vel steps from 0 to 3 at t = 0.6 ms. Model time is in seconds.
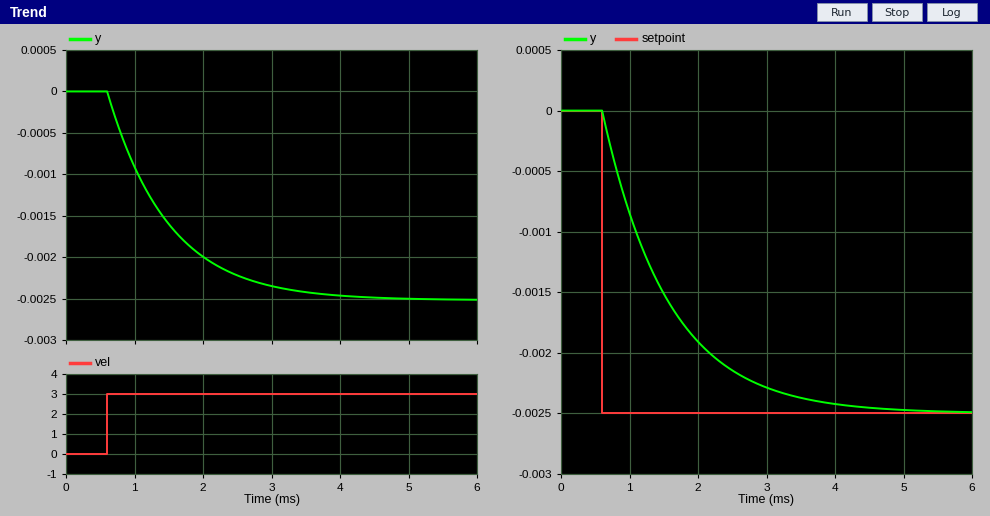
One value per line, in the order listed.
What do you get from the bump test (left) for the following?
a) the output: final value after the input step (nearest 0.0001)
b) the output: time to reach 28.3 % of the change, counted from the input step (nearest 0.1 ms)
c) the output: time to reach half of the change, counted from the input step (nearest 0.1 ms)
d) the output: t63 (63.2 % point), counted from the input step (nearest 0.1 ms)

-0.0025
0.3 ms
0.6 ms
0.9 ms
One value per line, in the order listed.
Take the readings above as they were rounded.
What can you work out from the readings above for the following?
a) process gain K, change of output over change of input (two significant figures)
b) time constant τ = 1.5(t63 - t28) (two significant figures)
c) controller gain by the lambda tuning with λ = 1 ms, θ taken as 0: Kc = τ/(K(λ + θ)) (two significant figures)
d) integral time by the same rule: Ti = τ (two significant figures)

-0.00083
0.90 ms
-1100
0.90 ms
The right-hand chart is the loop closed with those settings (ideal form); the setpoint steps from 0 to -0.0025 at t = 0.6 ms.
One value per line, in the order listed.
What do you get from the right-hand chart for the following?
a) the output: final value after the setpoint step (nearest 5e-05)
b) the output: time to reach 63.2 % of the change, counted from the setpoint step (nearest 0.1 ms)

-0.00250
1.0 ms
